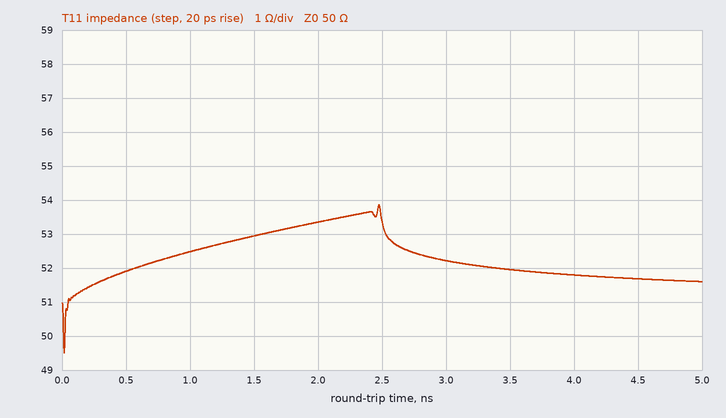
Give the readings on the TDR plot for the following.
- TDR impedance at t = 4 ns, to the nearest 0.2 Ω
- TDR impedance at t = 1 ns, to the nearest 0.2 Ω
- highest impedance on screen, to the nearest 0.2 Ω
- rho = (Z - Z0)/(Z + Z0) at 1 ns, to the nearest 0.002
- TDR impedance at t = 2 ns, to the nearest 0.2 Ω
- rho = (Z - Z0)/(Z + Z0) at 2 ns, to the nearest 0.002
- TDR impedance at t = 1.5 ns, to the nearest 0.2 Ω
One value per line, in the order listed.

51.8 Ω
52.4 Ω
53.8 Ω
+0.024
53.4 Ω
+0.032
53.0 Ω
